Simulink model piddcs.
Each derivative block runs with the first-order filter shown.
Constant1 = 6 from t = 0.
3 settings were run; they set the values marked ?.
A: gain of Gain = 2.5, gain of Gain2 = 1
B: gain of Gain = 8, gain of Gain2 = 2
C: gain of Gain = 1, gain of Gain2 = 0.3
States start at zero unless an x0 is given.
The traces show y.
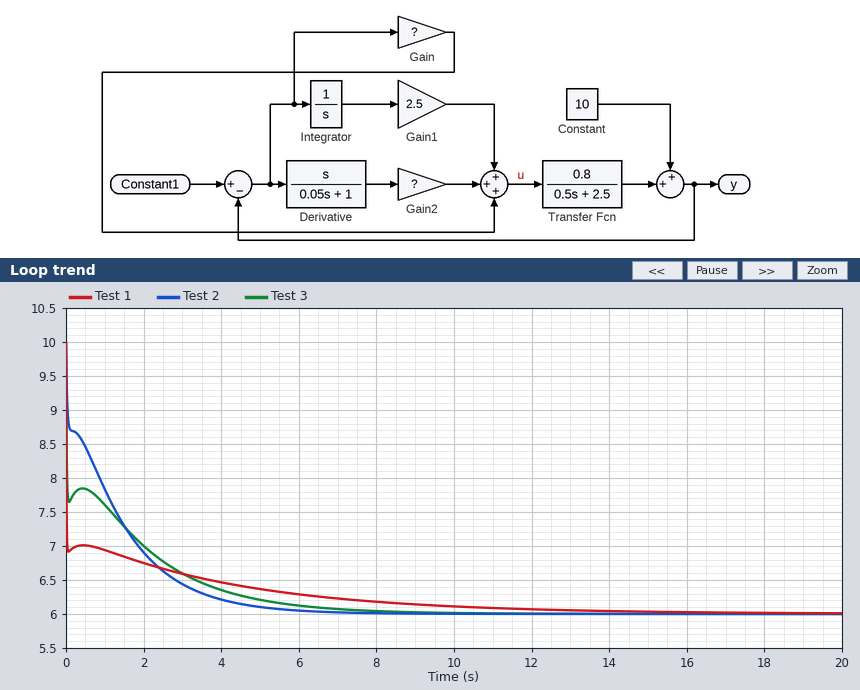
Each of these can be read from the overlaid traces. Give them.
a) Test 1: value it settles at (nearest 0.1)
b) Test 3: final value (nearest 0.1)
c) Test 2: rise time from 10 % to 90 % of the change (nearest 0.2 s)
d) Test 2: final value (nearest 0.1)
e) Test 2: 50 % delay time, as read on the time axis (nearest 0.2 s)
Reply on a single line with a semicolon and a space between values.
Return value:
6.0; 6.0; 3.2 s; 6.0; 0.8 s
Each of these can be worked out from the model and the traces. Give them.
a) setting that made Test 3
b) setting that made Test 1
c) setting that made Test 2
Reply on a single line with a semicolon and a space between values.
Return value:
A; B; C
